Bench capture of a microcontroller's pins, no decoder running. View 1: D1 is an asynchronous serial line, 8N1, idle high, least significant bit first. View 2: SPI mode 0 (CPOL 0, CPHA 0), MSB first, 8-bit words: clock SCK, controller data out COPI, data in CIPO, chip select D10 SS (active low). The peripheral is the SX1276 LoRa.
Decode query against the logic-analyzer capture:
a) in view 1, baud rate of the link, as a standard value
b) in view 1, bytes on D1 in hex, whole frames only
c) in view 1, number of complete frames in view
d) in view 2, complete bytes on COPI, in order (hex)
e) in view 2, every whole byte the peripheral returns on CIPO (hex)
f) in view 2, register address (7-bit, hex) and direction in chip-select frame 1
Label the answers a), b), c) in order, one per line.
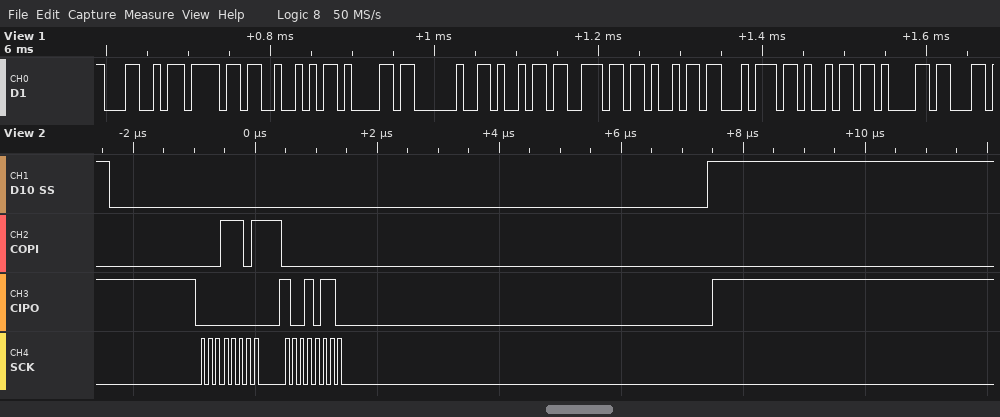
a) 115200 baud
b) 0x4C 0x6F 0x52 0x61 0x20 0x69 0x6E 0x69 0x74 0x69 0x61
c) 11
d) 1D 00
e) 00 96
f) 0x1D read
